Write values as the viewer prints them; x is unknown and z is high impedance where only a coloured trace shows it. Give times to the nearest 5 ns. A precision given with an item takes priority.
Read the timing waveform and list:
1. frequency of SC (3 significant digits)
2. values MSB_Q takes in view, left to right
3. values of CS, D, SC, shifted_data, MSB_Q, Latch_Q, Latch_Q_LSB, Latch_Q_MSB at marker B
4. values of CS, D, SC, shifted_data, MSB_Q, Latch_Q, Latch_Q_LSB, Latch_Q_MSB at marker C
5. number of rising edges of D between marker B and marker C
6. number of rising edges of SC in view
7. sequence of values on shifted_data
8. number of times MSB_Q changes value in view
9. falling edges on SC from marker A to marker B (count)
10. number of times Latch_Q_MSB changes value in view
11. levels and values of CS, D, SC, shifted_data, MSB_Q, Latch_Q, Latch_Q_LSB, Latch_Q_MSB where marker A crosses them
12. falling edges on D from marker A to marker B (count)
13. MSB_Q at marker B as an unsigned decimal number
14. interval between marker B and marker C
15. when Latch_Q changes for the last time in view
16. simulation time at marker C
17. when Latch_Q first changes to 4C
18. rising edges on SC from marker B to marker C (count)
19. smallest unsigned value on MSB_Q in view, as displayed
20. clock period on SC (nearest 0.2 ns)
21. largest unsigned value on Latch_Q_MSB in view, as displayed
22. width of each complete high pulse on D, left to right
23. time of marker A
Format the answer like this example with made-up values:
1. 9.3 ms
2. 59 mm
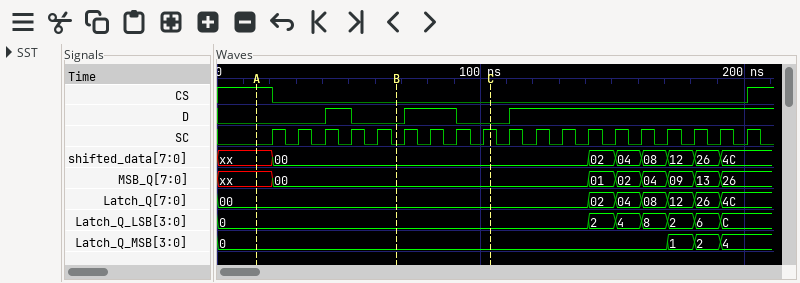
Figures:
1. 100 MHz
2. xx, 00, 01, 02, 04, 09, 13, 26
3. CS=0, D=0, SC=0, shifted_data=00, MSB_Q=00, Latch_Q=00, Latch_Q_LSB=0, Latch_Q_MSB=0
4. CS=0, D=0, SC=1, shifted_data=00, MSB_Q=00, Latch_Q=00, Latch_Q_LSB=0, Latch_Q_MSB=0
5. 1
6. 19
7. xx, 00, 02, 04, 08, 12, 26, 4C
8. 7
9. 5
10. 3
11. CS=1, D=0, SC=0, shifted_data=xx, MSB_Q=xx, Latch_Q=00, Latch_Q_LSB=0, Latch_Q_MSB=0
12. 1
13. 0
14. 35 ns
15. 190 ns
16. 105 ns
17. 190 ns
18. 4
19. 00
20. 10 ns
21. 4
22. 10 ns, 20 ns
23. 15 ns
